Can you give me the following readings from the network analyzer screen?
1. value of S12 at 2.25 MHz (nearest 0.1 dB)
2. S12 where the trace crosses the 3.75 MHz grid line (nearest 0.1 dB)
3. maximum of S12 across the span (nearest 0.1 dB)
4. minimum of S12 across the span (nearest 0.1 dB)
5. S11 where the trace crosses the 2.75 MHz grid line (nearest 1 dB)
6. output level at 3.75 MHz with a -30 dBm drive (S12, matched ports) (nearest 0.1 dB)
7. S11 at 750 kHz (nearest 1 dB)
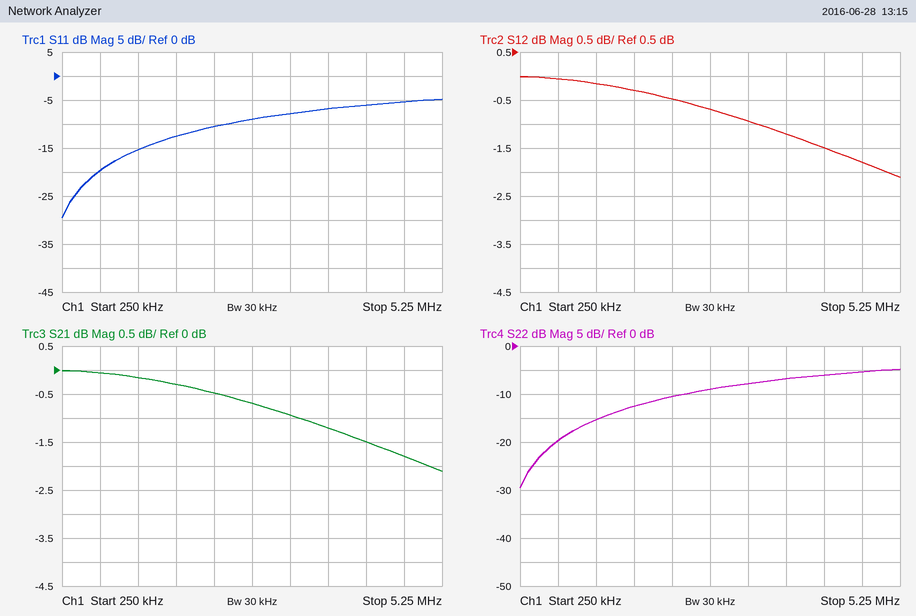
-0.5 dB
-1.2 dB
0.0 dB
-2.1 dB
-9 dB
-31.2 dBm
-20 dB
